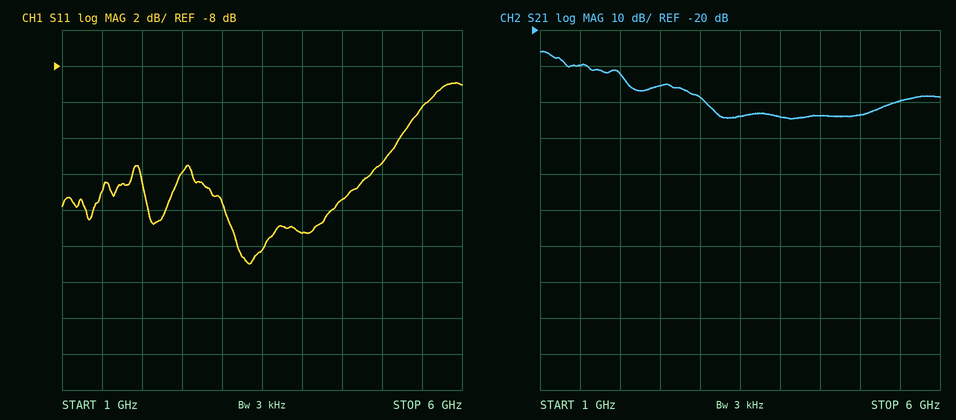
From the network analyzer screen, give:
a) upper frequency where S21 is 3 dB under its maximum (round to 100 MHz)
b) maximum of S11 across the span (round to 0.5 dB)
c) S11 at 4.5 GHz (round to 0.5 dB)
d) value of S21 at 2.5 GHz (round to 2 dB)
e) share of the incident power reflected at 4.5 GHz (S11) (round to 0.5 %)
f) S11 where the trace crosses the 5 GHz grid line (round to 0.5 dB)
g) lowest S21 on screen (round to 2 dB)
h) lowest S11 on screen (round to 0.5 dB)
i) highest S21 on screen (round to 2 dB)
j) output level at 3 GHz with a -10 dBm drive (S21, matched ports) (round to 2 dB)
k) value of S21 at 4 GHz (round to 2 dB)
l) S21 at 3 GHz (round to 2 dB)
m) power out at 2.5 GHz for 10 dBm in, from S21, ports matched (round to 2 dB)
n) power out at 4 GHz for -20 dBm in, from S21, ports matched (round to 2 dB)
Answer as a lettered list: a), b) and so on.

a) 1.3 GHz
b) -9.0 dB
c) -15.5 dB
d) -36 dB
e) 3.0 %
f) -13.5 dB
g) -44 dB
h) -19.0 dB
i) -26 dB
j) -48 dBm
k) -44 dB
l) -38 dB
m) -26 dBm
n) -64 dBm
